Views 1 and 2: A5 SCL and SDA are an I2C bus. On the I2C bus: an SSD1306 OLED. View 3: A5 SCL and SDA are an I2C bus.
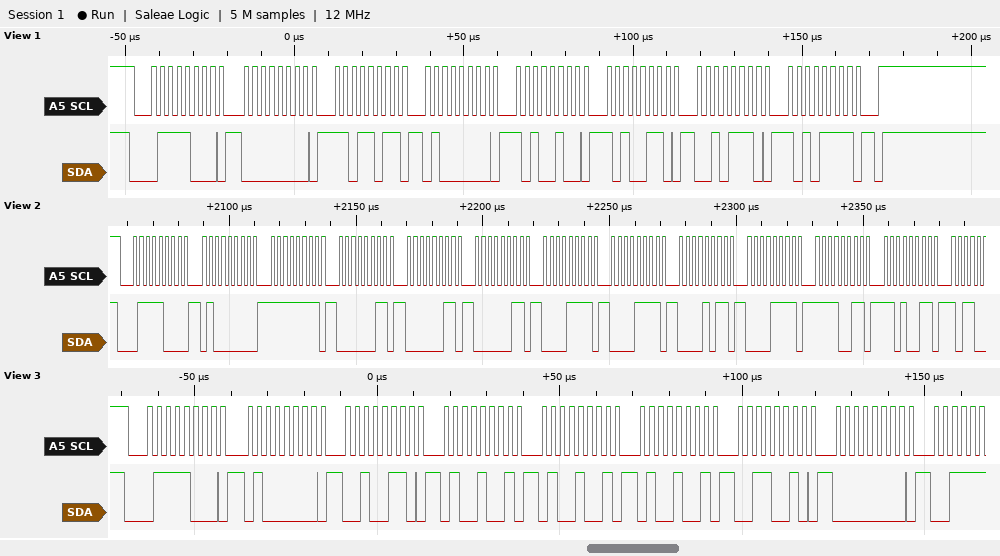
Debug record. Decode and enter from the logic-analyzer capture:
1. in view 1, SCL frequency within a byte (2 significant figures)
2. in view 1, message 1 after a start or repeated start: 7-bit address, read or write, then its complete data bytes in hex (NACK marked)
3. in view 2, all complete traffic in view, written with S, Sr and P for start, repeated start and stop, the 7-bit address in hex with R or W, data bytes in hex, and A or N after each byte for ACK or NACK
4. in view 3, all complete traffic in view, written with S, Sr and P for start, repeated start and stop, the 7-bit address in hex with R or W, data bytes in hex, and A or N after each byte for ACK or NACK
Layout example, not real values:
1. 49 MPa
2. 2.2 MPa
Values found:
1. 400 kHz
2. 0x3C write: 00 DB 40 A4 A6 2E AF
3. S 3CW A 40 A FF A 03 A 03 A 03 A 0F A 0F A 0B A 0F A F3 A D3 A
4. S 3CW A 40 A 26 A 49 A 49 A 49 A 32 A 00 A
